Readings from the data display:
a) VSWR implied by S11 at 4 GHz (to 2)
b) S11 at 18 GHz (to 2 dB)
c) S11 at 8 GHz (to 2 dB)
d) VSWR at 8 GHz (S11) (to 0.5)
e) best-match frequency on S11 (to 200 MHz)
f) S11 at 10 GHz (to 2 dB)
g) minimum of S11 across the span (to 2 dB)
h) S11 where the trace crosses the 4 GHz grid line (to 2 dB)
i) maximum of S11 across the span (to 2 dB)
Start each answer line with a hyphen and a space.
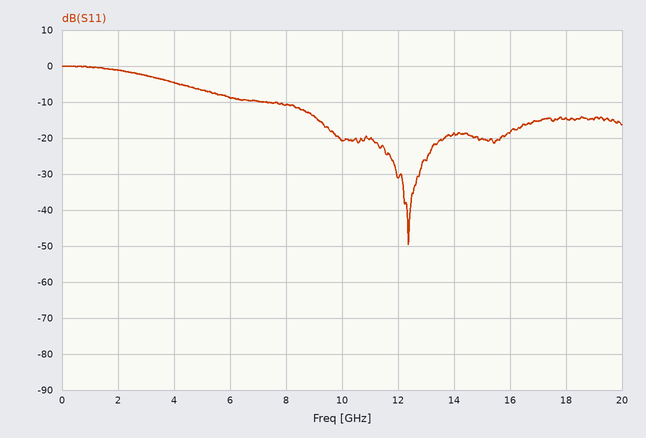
- 4
- -14 dB
- -10 dB
- 2.0
- 12.4 GHz
- -20 dB
- -50 dB
- -4 dB
- 0 dB
